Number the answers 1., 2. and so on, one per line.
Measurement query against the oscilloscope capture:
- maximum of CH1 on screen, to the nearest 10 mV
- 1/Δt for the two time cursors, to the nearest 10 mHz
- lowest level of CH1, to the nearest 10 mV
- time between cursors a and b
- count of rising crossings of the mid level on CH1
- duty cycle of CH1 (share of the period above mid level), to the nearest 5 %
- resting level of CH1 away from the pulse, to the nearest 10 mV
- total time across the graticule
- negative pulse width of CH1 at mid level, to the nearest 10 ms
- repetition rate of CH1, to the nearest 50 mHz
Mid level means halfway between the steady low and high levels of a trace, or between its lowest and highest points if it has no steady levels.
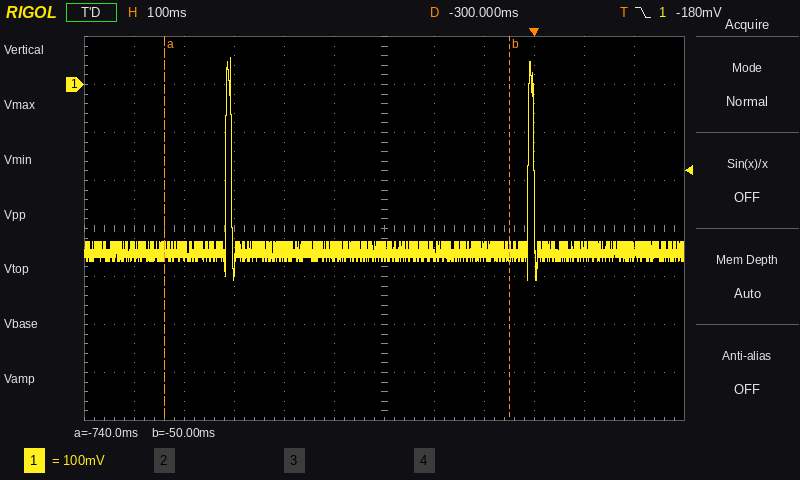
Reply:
1. 60 mV
2. 1.45 Hz
3. -410 mV
4. 690 ms
5. 2
6. 0 %
7. -350 mV
8. 1.2 s
9. 590 ms
10. 1.65 Hz
